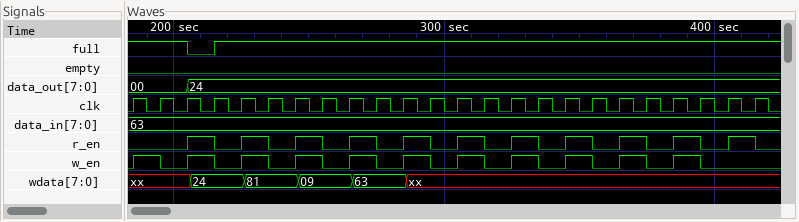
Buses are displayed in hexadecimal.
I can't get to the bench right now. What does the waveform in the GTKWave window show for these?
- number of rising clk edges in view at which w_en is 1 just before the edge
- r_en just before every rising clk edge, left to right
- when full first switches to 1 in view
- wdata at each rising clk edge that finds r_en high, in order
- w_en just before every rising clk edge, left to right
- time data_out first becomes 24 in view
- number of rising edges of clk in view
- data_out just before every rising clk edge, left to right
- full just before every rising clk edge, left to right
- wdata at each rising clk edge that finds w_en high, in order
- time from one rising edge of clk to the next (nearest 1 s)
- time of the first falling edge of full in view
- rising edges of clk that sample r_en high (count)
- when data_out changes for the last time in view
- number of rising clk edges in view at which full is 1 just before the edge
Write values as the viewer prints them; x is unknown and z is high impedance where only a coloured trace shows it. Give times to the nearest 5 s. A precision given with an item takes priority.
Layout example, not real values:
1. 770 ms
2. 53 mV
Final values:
1. 11
2. 0 0 0 1 0 1 0 1 0 1 0 1 0 1 0 1 0 1 0 1 0 1 0 1
3. 215 s
4. 24, 81, 09, 63, xx, xx, xx, xx, xx, xx, xx
5. 0 1 0 1 0 1 0 1 0 1 0 1 0 1 0 1 0 1 0 1 0 1 0 0
6. 205 s
7. 24
8. 00, 00, 00, 24, 24, 24, 24, 24, 24, 24, 24, 24, 24, 24, 24, 24, 24, 24, 24, 24, 24, 24, 24, 24
9. 1 1 1 0 1 1 1 1 1 1 1 1 1 1 1 1 1 1 1 1 1 1 1 1
10. xx, 24, 81, 09, 63, xx, xx, xx, xx, xx, xx
11. 10 s
12. 205 s
13. 11
14. 205 s
15. 23
